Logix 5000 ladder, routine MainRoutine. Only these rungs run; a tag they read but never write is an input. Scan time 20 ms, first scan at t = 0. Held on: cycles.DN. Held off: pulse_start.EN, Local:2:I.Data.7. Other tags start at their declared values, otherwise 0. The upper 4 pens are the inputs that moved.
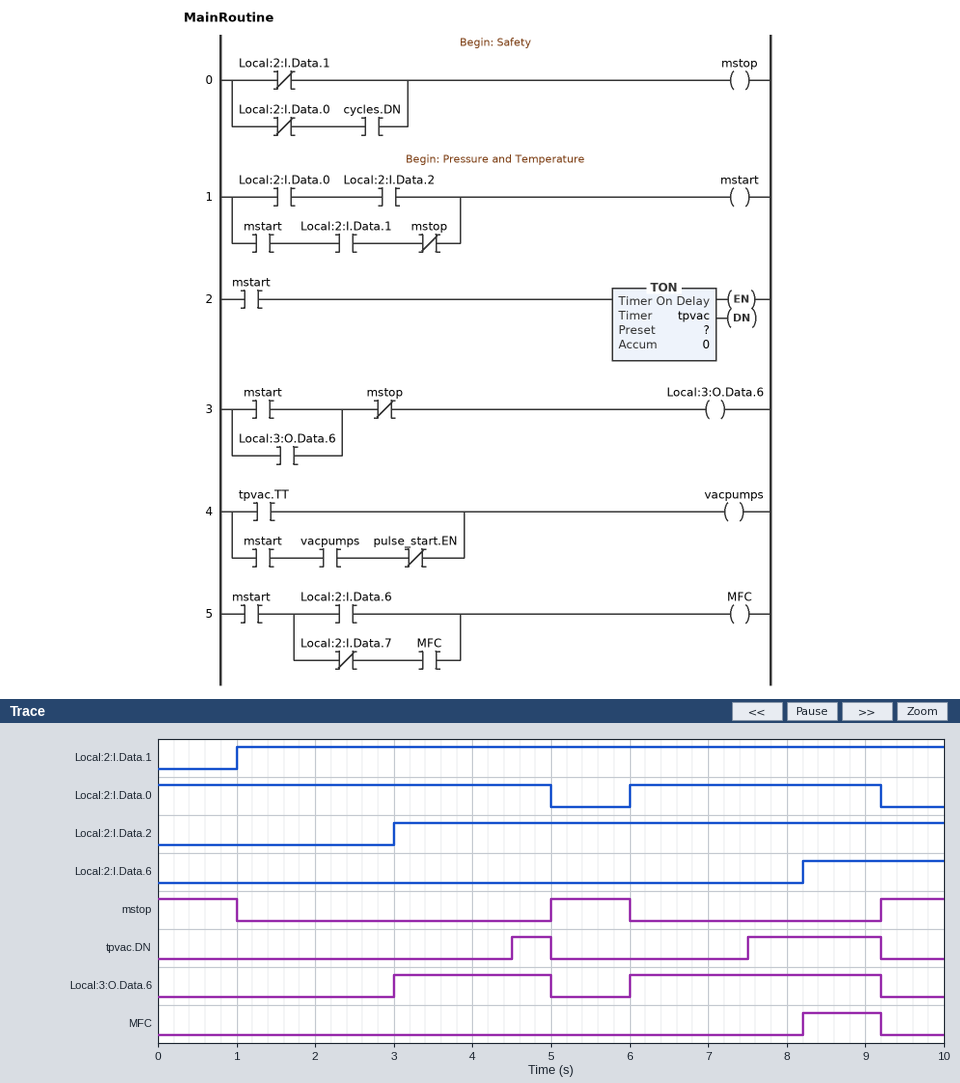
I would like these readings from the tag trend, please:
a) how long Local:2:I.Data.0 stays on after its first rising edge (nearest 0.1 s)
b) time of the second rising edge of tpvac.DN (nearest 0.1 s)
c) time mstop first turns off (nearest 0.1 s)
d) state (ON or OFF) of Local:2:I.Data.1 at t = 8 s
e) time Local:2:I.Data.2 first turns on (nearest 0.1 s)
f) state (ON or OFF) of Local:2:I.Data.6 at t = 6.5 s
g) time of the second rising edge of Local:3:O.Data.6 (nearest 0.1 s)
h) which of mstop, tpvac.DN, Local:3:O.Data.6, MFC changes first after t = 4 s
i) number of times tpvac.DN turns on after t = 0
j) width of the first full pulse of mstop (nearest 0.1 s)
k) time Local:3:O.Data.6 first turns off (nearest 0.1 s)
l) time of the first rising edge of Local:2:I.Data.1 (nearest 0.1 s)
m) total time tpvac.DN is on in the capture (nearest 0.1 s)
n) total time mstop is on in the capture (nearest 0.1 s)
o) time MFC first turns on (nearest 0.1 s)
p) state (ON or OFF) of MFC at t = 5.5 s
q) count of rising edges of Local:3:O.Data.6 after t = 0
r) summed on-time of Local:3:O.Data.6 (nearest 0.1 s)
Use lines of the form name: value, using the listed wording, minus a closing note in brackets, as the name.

how long Local:2:I.Data.0 stays on after its first rising edge: 3.2 s
time of the second rising edge of tpvac.DN: 7.5 s
time mstop first turns off: 1.0 s
state (ON or OFF) of Local:2:I.Data.1 at t = 8 s: ON
time Local:2:I.Data.2 first turns on: 3.0 s
state (ON or OFF) of Local:2:I.Data.6 at t = 6.5 s: OFF
time of the second rising edge of Local:3:O.Data.6: 6.0 s
which of mstop, tpvac.DN, Local:3:O.Data.6, MFC changes first after t = 4 s: tpvac.DN
number of times tpvac.DN turns on after t = 0: 2
width of the first full pulse of mstop: 1.0 s
time Local:3:O.Data.6 first turns off: 5.0 s
time of the first rising edge of Local:2:I.Data.1: 1.0 s
total time tpvac.DN is on in the capture: 2.2 s
total time mstop is on in the capture: 2.8 s
time MFC first turns on: 8.2 s
state (ON or OFF) of MFC at t = 5.5 s: OFF
count of rising edges of Local:3:O.Data.6 after t = 0: 2
summed on-time of Local:3:O.Data.6: 5.2 s
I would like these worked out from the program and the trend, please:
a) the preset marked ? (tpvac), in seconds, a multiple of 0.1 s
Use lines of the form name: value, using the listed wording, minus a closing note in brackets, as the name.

the preset marked ? (tpvac), in seconds, a multiple of 0.1 s: 1.5 s
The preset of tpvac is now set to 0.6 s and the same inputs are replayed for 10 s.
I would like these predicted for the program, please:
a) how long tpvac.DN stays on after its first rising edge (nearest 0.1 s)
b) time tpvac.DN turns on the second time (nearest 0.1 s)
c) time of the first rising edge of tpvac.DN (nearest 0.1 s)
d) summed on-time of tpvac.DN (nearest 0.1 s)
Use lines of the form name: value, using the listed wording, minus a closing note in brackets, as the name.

how long tpvac.DN stays on after its first rising edge: 1.4 s
time tpvac.DN turns on the second time: 6.6 s
time of the first rising edge of tpvac.DN: 3.6 s
summed on-time of tpvac.DN: 4.0 s
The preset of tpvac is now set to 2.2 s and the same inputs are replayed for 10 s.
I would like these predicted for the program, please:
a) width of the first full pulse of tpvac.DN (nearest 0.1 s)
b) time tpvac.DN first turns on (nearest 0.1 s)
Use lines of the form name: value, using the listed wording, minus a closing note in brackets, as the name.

width of the first full pulse of tpvac.DN: 1.0 s
time tpvac.DN first turns on: 8.2 s
